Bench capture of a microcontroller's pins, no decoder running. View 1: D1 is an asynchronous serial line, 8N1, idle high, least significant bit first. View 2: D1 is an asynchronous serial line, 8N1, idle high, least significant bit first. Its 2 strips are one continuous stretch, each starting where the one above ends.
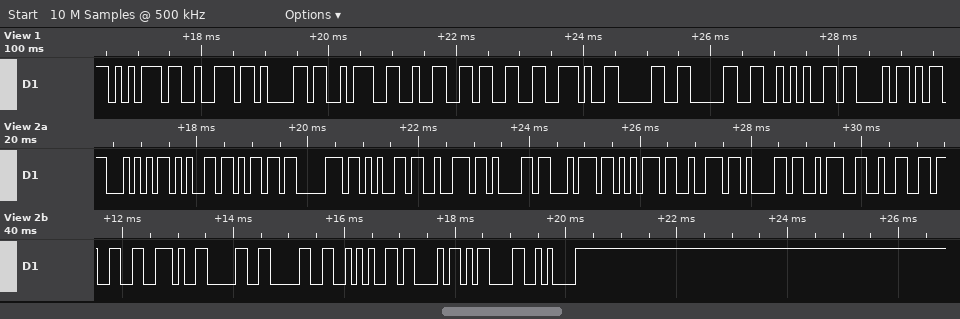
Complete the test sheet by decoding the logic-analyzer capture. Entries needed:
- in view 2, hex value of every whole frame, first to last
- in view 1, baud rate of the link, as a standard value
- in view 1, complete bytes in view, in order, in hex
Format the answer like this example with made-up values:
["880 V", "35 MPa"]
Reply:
["0x54 0x65 0x6D 0x70 0x65 0x72 0x61 0x74 0x75 0x72 0x61 0x3A 0x32 0x33 0x2E 0x30 0x30 0x2A 0x43 0x0D 0x0A", "9600 baud", "75 72 61 3A 32 33 2E 30 30 2A 43"]
